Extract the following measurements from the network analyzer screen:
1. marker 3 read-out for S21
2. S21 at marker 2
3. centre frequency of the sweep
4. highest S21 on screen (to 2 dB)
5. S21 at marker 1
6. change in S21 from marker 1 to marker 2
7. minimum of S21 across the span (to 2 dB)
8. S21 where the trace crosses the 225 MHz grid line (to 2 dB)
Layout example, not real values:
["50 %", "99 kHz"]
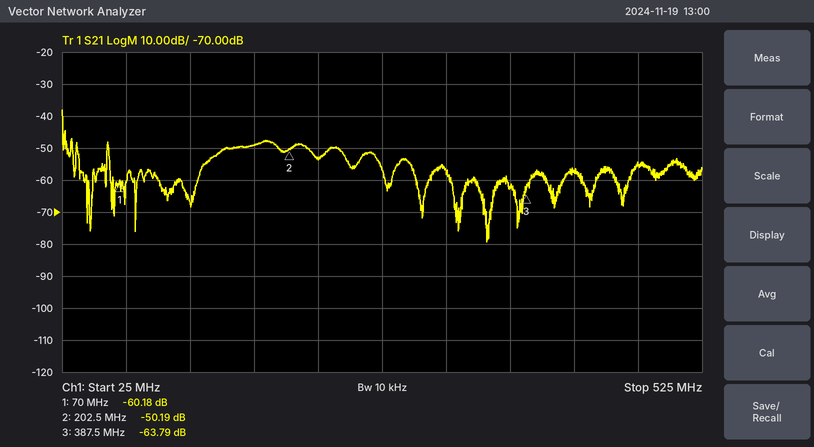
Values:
["-63.79 dB", "-50.19 dB", "275 MHz", "-38 dB", "-60.18 dB", "9.99 dB", "-80 dB", "-54 dB"]
